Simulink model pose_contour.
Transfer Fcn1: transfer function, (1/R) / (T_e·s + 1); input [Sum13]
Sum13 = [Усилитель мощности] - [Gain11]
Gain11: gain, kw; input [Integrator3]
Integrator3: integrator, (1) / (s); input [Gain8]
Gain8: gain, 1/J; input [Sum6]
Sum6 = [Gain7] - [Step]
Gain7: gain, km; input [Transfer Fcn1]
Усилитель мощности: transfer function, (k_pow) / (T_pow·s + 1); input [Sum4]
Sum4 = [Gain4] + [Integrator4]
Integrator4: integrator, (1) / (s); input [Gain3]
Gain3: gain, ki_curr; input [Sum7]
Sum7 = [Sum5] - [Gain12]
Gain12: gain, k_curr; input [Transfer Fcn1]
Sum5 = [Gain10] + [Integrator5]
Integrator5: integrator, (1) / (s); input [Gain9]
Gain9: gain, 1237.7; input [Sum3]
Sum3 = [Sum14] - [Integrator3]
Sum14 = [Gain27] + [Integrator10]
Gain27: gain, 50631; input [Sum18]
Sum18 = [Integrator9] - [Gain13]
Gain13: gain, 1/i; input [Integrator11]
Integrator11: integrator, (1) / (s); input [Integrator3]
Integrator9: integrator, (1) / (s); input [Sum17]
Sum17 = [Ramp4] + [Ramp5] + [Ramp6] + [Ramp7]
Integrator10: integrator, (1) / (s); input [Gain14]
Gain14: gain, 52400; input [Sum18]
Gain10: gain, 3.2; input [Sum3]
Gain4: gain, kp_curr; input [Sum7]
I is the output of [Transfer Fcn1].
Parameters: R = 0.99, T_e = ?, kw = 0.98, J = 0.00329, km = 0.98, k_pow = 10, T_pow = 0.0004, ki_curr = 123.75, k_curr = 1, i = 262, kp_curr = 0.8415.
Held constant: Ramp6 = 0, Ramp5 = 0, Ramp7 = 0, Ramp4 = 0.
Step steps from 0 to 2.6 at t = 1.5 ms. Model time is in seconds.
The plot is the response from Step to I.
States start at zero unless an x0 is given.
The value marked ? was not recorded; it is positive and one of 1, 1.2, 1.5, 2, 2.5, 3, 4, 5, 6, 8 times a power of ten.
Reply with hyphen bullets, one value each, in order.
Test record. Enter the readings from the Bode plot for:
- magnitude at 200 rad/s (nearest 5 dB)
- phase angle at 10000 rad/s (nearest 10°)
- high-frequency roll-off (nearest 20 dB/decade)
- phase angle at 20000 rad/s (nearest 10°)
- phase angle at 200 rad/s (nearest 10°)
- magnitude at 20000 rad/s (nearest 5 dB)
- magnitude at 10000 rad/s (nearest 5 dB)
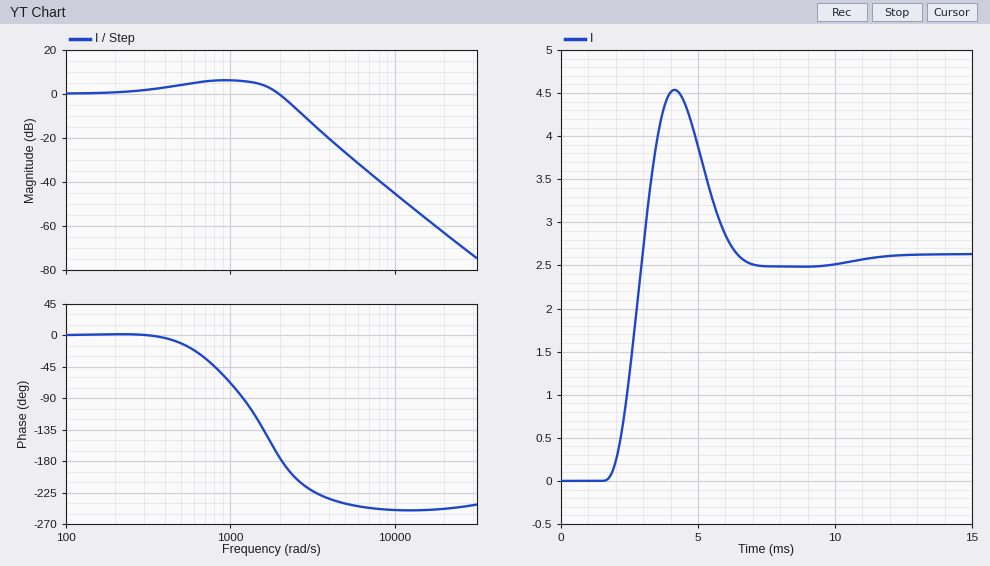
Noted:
- 0 dB
- -250°
- -60 dB/decade
- -250°
- 0°
- -65 dB
- -45 dB
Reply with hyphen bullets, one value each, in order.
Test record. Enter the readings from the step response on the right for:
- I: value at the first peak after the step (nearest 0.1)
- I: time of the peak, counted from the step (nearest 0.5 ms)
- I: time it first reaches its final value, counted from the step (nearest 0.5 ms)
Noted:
- 4.5
- 2.5 ms
- 1.5 ms
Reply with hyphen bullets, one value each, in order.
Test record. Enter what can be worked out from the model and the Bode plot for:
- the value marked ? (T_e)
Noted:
- 0.004
